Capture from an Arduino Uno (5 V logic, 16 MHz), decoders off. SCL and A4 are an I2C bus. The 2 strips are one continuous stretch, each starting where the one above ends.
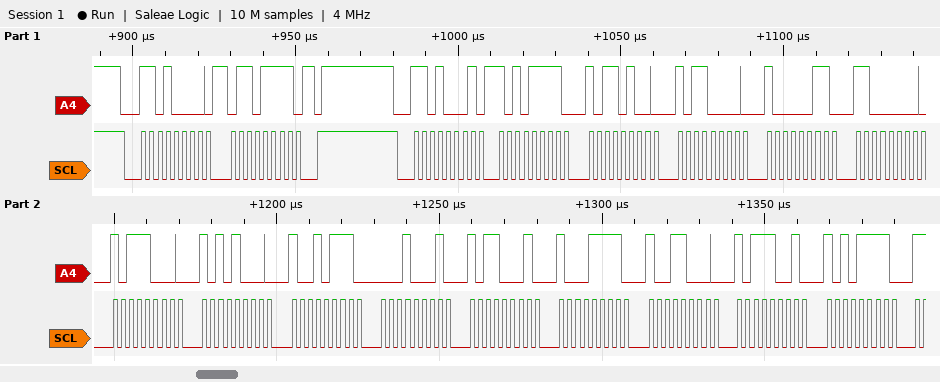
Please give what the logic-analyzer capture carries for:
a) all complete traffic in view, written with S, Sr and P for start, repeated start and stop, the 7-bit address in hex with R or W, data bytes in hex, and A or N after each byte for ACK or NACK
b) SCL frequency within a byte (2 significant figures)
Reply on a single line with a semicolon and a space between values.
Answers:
S 68W A 6F A P S 68R A AF A B4 A B0 A 83 A C0 A B8 A A8 A 97 A 11 A B1 A 8F A 98 A B9 A AF A; 400 kHz
